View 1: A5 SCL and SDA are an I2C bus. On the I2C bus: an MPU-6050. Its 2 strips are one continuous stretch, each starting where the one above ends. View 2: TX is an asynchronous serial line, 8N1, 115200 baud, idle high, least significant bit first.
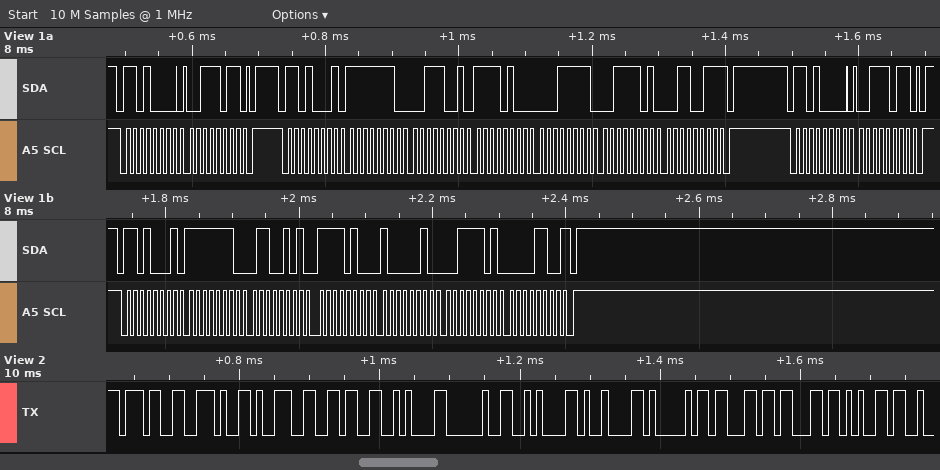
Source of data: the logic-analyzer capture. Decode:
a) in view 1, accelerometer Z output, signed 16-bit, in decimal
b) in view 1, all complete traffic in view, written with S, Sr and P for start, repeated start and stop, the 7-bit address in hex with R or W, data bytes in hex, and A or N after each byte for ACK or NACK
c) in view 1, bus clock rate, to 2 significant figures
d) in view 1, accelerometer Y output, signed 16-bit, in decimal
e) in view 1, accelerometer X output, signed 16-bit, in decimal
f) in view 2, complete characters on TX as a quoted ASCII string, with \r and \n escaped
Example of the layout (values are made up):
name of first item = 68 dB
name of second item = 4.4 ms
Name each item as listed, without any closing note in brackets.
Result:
in view 1, accelerometer Z output, signed 16-bit, in decimal = 15667
in view 1, all complete traffic in view, written with S, Sr and P for start, repeated start and stop, the 7-bit address in hex with R or W, data bytes in hex, and A or N after each byte for ACK or NACK = S 68W A 3B A P S 68R A FE A 39 A F4 A 1F A 3D A 33 N P S 68W A 3B A P S 68R A FE A 65 A F4 A 82 A 3D A 0C N P
in view 1, bus clock rate, to 2 significant figures = 100 kHz
in view 1, accelerometer Y output, signed 16-bit, in decimal = -3041
in view 1, accelerometer X output, signed 16-bit, in decimal = -455
in view 2, complete characters on TX as a quoted ASCII string, with \r and \n escaped = "7.96\n \n\tAcce"
